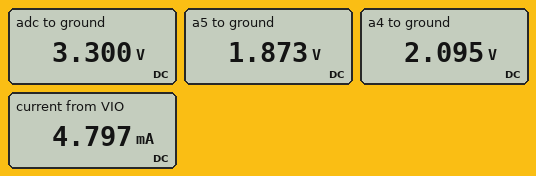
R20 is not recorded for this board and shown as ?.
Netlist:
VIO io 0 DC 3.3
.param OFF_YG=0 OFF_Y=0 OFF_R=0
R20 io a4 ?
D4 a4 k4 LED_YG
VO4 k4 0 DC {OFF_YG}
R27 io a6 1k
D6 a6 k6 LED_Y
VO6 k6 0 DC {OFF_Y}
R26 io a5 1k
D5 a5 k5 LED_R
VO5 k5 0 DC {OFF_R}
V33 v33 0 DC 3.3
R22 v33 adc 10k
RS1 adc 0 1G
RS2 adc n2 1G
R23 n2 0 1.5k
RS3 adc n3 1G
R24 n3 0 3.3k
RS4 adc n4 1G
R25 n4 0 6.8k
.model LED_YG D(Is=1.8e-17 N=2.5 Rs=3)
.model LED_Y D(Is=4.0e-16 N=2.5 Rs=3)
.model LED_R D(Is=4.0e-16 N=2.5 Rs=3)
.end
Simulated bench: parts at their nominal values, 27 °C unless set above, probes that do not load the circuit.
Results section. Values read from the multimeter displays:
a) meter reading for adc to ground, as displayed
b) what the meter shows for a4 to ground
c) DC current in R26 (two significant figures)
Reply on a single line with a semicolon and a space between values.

3.300 V; 2.095 V; 1.4 mA
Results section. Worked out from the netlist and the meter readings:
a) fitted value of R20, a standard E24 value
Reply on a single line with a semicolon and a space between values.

620 Ω
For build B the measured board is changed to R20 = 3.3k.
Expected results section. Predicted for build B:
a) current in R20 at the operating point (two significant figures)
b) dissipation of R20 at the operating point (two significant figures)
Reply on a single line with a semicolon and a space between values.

400 µA; 520 µW
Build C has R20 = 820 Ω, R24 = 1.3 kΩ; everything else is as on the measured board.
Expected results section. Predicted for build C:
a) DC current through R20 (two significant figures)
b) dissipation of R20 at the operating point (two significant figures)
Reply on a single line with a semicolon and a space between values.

1.5 mA; 1.8 mW
